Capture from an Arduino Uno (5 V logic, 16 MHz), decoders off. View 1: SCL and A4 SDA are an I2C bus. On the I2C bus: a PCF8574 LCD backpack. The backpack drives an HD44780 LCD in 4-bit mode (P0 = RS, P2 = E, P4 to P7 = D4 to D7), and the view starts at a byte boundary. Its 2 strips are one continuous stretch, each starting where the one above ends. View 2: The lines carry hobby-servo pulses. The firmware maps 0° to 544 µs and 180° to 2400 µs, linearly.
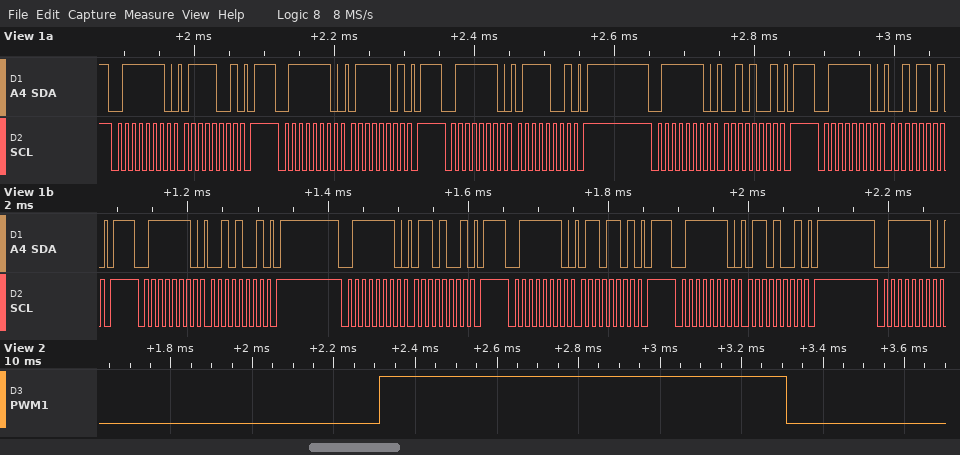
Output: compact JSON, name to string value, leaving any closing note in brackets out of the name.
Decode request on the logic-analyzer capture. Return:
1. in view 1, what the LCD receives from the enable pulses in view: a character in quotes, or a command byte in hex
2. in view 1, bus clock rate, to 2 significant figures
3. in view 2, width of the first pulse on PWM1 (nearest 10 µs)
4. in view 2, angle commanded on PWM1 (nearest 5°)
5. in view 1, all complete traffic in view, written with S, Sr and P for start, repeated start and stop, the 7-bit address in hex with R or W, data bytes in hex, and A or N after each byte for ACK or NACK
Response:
{"in view 1, what the LCD receives from the enable pulses in view: a character in quotes, or a command byte in hex": "'r'", "in view 1, bus clock rate, to 2 significant figures": "100 kHz", "in view 2, width of the first pulse on PWM1": "1000 µs", "in view 2, angle commanded on PWM1": "45°", "in view 1, all complete traffic in view, written with S, Sr and P for start, repeated start and stop, the 7-bit address in hex with R or W, data bytes in hex, and A or N after each byte for ACK or NACK": "S 3FW A 79 A P S 3FW A 7D A P S 3FW A 79 A P S 3FW A 29 A P S 3FW A 2D A P S 3FW A 29 A P S 3FW A 69 A P S 3FW A 6D A P S 3FW A 69 A P S 3FW A"}
